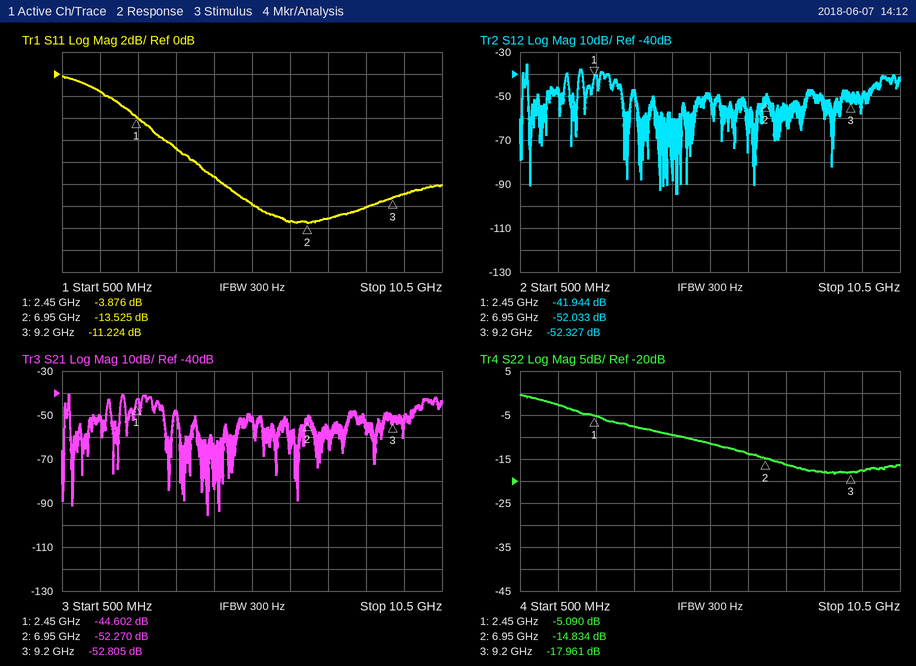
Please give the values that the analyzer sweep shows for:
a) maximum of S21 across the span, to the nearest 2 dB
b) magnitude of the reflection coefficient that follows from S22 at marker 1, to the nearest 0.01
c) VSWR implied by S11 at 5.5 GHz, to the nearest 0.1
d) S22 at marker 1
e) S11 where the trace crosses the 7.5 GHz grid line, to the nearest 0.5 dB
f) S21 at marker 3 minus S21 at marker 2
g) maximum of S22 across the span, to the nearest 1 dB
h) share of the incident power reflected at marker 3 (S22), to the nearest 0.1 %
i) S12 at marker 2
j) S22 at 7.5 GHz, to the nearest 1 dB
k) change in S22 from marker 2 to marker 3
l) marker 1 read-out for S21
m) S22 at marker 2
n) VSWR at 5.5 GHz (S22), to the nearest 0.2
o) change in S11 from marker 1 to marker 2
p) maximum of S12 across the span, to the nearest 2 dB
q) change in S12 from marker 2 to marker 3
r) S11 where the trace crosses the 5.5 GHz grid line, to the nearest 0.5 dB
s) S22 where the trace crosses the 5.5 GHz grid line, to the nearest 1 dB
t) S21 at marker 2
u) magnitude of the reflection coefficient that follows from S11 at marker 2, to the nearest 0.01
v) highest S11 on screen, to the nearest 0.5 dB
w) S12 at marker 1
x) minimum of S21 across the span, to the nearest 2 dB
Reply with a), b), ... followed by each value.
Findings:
a) -40 dB
b) 0.56
c) 1.7
d) -5.090 dB
e) -13.0 dB
f) -0.535 dB
g) 0 dB
h) 1.6 %
i) -52.033 dB
j) -16 dB
k) -3.127 dB
l) -44.602 dB
m) -14.834 dB
n) 1.8
o) -9.649 dB
p) -36 dB
q) -0.294 dB
r) -12.0 dB
s) -11 dB
t) -52.270 dB
u) 0.21
v) 0.0 dB
w) -41.944 dB
x) -96 dB
